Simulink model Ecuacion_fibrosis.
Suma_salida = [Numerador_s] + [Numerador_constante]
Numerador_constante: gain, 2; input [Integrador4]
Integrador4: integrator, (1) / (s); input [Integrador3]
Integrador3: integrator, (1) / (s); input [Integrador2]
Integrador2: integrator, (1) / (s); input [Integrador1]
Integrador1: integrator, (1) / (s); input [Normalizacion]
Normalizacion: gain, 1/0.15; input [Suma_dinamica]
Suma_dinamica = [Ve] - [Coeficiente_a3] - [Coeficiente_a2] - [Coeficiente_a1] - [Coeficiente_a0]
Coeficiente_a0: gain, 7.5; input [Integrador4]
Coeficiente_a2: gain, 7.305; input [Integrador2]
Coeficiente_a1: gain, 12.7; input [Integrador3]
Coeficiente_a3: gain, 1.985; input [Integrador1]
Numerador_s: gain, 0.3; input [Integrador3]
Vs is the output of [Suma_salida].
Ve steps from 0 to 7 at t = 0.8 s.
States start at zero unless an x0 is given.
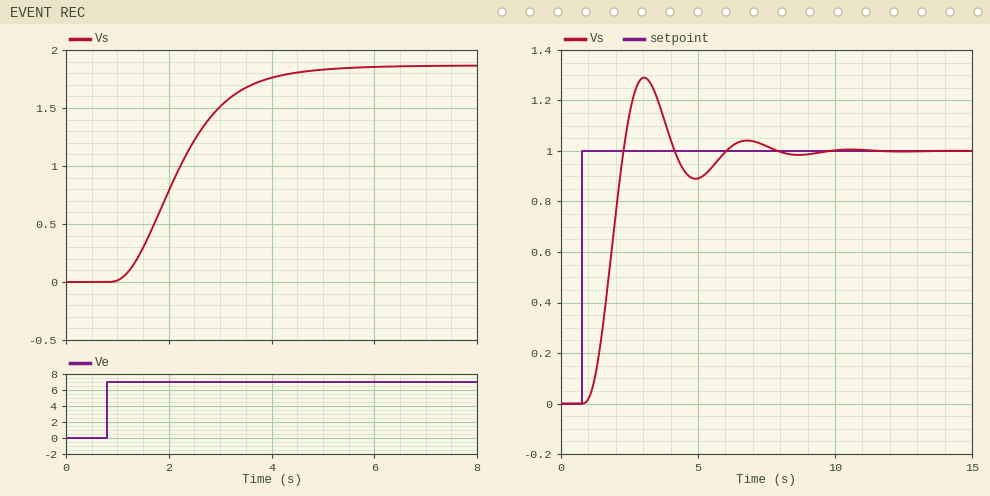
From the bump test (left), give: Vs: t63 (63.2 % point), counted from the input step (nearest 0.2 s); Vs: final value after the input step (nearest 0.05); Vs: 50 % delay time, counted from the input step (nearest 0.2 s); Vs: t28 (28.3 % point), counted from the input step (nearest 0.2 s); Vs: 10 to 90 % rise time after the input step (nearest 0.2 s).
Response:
1.6 s
1.85
1.4 s
1.0 s
2.2 s
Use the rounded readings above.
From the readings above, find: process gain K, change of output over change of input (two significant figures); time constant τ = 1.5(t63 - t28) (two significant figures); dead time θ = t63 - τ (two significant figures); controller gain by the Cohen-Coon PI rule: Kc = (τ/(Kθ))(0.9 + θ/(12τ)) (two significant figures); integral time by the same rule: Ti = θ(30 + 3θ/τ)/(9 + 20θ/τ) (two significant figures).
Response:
0.26
0.90 s
0.70 s
4.8
0.92 s
